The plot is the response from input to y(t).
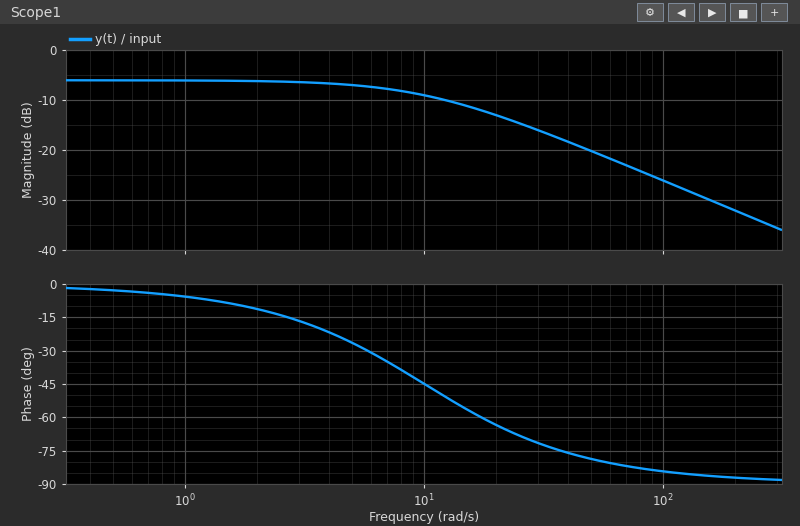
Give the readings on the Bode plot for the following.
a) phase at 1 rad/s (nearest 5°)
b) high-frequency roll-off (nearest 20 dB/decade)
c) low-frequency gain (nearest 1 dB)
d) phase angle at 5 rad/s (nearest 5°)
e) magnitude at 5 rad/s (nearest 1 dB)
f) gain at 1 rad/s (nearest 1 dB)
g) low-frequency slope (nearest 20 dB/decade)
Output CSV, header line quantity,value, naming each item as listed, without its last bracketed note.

quantity,value
phase at 1 rad/s,-5°
high-frequency roll-off,-20 dB/decade
low-frequency gain,-6 dB
phase angle at 5 rad/s,-25°
magnitude at 5 rad/s,-7 dB
gain at 1 rad/s,-6 dB
low-frequency slope,0 dB/decade
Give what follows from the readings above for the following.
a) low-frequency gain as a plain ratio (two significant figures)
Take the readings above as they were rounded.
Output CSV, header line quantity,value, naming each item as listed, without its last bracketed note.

quantity,value
low-frequency gain as a plain ratio,0.50
